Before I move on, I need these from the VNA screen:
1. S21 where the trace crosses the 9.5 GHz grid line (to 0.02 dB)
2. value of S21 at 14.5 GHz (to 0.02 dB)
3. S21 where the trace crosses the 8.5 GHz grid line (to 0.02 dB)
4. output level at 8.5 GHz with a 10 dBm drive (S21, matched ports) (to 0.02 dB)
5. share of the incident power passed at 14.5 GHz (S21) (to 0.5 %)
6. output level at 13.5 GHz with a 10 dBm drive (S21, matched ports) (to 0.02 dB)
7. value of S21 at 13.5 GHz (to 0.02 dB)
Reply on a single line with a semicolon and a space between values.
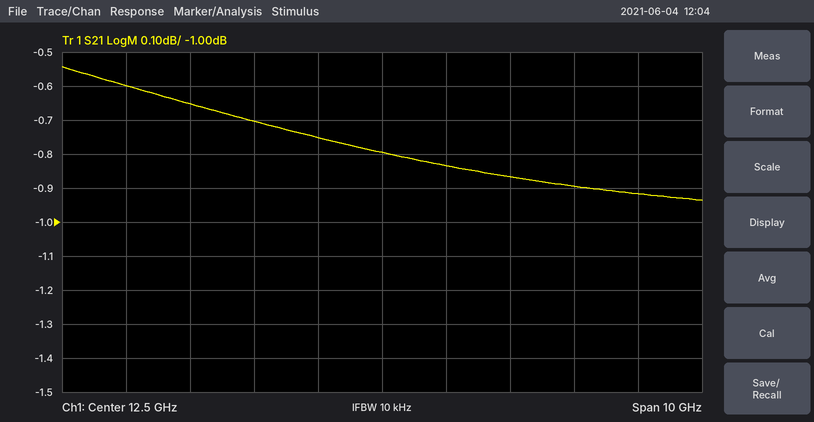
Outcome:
-0.66 dB; -0.86 dB; -0.60 dB; 9.40 dBm; 82.0 %; 9.16 dBm; -0.84 dB
